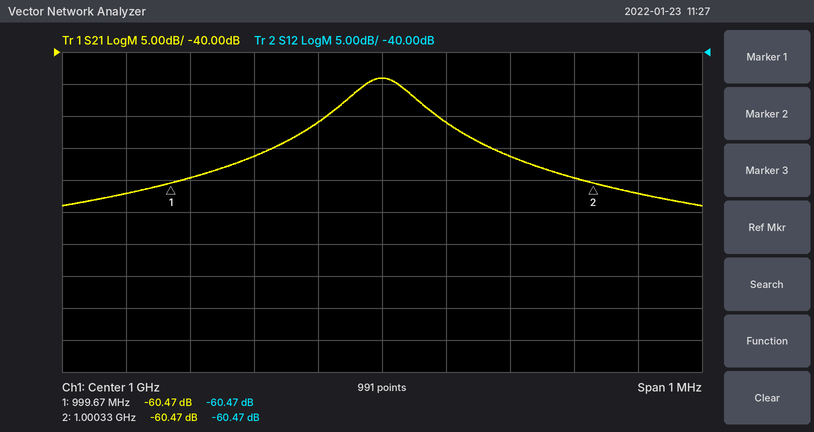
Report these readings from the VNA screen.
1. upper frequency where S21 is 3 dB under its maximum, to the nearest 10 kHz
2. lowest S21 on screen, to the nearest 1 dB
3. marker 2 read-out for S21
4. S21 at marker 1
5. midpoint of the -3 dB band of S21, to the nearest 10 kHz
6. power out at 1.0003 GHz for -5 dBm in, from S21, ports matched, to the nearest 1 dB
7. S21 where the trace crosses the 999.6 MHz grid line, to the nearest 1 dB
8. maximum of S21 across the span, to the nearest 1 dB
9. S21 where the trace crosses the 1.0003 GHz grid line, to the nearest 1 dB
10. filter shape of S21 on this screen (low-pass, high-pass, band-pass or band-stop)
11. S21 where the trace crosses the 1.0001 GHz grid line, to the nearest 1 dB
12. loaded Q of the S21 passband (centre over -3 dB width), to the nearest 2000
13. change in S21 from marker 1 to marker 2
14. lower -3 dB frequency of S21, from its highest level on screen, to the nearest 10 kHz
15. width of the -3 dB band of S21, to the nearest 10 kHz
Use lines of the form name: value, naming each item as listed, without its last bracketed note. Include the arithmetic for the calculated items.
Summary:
upper frequency where S21 is 3 dB under its maximum, to the nearest 10 kHz: 1.00005 GHz
lowest S21 on screen, to the nearest 1 dB: -64 dB
marker 2 read-out for S21: -60.47 dB
S21 at marker 1: -60.47 dB
midpoint of the -3 dB band of S21, to the nearest 10 kHz: 1.00000 GHz
power out at 1.0003 GHz for -5 dBm in, from S21, ports matched, to the nearest 1 dB: -5 dBm + (-60 dB) = -65 dBm
S21 where the trace crosses the 999.6 MHz grid line, to the nearest 1 dB: -62 dB
maximum of S21 across the span, to the nearest 1 dB: -44 dB
S21 where the trace crosses the 1.0003 GHz grid line, to the nearest 1 dB: -60 dB
filter shape of S21 on this screen: band-pass
S21 where the trace crosses the 1.0001 GHz grid line, to the nearest 1 dB: -51 dB
loaded Q of the S21 passband (centre over -3 dB width), to the nearest 2000: 1 GHz / 100 kHz ≈ 10000
change in S21 from marker 1 to marker 2: -60.47 − (-60.47) = 0.00 dB
lower -3 dB frequency of S21, from its highest level on screen, to the nearest 10 kHz: 999.95 MHz
width of the -3 dB band of S21, to the nearest 10 kHz: 1.00005 GHz − 999.95 MHz = 100 kHz
